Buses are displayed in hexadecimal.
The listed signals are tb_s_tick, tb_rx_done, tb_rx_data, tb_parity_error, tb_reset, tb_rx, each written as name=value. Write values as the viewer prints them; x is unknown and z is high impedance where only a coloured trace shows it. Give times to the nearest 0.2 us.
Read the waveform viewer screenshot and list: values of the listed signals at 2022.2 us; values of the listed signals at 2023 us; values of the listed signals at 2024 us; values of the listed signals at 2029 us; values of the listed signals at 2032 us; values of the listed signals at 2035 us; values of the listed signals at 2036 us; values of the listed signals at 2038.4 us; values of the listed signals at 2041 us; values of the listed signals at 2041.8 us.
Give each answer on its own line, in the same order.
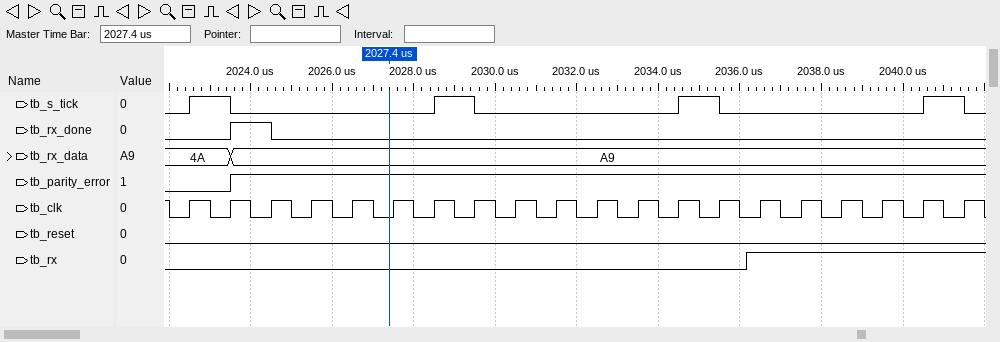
tb_s_tick=0, tb_rx_done=0, tb_rx_data=4A, tb_parity_error=0, tb_reset=0, tb_rx=0
tb_s_tick=1, tb_rx_done=0, tb_rx_data=4A, tb_parity_error=0, tb_reset=0, tb_rx=0
tb_s_tick=0, tb_rx_done=1, tb_rx_data=A9, tb_parity_error=1, tb_reset=0, tb_rx=0
tb_s_tick=1, tb_rx_done=0, tb_rx_data=A9, tb_parity_error=1, tb_reset=0, tb_rx=0
tb_s_tick=0, tb_rx_done=0, tb_rx_data=A9, tb_parity_error=1, tb_reset=0, tb_rx=0
tb_s_tick=1, tb_rx_done=0, tb_rx_data=A9, tb_parity_error=1, tb_reset=0, tb_rx=0
tb_s_tick=0, tb_rx_done=0, tb_rx_data=A9, tb_parity_error=1, tb_reset=0, tb_rx=0
tb_s_tick=0, tb_rx_done=0, tb_rx_data=A9, tb_parity_error=1, tb_reset=0, tb_rx=1
tb_s_tick=1, tb_rx_done=0, tb_rx_data=A9, tb_parity_error=1, tb_reset=0, tb_rx=1
tb_s_tick=0, tb_rx_done=0, tb_rx_data=A9, tb_parity_error=1, tb_reset=0, tb_rx=1
